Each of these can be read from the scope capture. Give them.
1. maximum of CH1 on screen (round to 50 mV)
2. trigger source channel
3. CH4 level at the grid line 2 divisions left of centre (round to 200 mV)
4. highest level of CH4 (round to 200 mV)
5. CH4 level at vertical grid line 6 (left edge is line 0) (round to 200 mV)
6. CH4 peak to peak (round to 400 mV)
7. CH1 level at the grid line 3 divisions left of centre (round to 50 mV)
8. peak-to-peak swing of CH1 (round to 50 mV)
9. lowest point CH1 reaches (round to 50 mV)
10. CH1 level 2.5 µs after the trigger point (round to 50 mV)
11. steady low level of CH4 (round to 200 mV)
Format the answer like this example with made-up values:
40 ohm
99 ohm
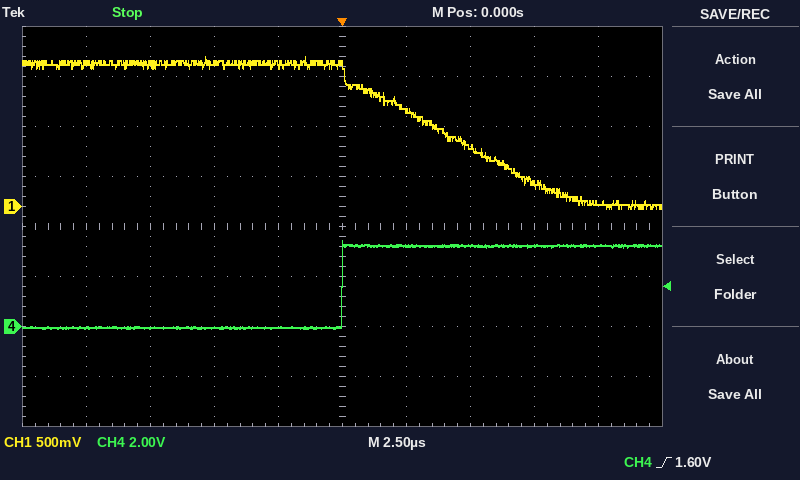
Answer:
1.50 V
CH4
0.0 V
3.4 V
3.2 V
3.6 V
1.40 V
1.50 V
0 mV
950 mV
0.0 V
